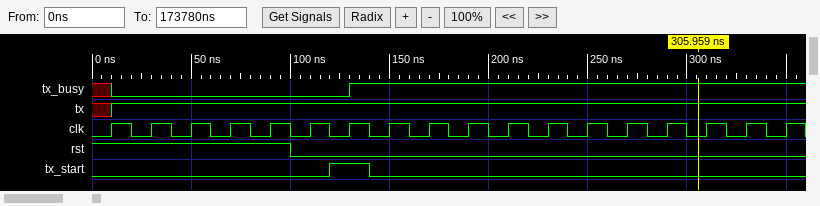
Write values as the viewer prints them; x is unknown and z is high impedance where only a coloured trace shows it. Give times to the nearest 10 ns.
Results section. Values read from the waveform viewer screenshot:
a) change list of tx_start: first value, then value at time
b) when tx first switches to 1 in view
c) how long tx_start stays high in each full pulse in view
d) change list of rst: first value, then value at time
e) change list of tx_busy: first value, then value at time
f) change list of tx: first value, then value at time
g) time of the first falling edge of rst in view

0, 1 at 120 ns, 0 at 140 ns
10 ns
20 ns
1, 0 at 100 ns
x, 0 at 10 ns, 1 at 130 ns
x, 1 at 10 ns
100 ns
